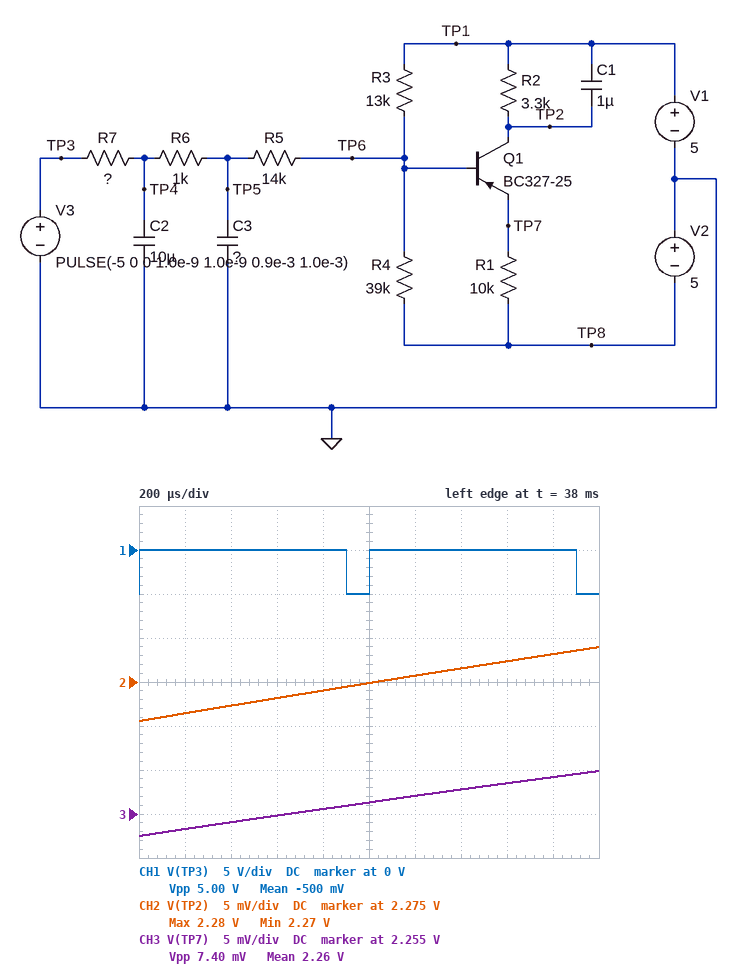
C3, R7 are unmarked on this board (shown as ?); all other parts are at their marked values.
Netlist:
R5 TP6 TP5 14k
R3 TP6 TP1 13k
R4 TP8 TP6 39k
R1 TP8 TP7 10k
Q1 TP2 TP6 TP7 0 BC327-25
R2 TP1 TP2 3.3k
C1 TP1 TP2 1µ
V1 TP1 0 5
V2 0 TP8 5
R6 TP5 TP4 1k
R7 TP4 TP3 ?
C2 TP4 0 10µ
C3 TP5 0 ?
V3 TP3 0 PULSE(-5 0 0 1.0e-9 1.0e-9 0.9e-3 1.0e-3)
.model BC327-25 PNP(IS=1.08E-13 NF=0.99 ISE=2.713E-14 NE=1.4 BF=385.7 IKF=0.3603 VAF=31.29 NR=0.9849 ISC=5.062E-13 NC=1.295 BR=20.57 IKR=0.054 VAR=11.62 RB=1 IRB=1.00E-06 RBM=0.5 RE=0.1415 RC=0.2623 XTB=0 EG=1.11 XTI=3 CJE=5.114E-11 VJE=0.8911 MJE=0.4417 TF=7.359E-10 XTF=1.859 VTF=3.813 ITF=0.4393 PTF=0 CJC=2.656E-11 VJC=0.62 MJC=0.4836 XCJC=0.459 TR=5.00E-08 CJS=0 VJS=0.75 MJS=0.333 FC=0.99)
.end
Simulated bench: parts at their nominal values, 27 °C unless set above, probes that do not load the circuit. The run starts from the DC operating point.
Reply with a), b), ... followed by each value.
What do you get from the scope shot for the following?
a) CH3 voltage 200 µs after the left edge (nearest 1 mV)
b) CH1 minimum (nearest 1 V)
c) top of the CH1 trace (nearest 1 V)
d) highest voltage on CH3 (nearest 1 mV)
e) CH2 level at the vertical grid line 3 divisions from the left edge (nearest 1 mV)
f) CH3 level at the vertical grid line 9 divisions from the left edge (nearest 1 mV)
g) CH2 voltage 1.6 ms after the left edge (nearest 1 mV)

a) 2.253 V
b) -5 V
c) 0 V
d) 2.260 V
e) 2.273 V
f) 2.259 V
g) 2.277 V
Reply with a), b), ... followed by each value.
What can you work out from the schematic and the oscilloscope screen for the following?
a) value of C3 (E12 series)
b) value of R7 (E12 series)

a) 12 µF
b) 470 Ω
